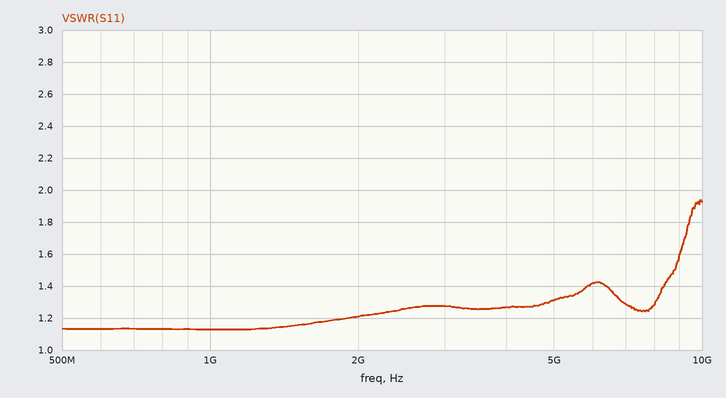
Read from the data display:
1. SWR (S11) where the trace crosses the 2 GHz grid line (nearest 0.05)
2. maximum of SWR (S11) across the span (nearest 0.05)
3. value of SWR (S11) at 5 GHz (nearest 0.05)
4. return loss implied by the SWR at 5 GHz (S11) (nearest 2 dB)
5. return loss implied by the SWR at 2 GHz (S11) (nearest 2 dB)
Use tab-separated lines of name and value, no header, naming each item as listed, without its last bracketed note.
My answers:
SWR (S11) where the trace crosses the 2 GHz grid line	1.20
maximum of SWR (S11) across the span	1.95
value of SWR (S11) at 5 GHz	1.30
return loss implied by the SWR at 5 GHz (S11)	18 dB
return loss implied by the SWR at 2 GHz (S11)	20 dB
